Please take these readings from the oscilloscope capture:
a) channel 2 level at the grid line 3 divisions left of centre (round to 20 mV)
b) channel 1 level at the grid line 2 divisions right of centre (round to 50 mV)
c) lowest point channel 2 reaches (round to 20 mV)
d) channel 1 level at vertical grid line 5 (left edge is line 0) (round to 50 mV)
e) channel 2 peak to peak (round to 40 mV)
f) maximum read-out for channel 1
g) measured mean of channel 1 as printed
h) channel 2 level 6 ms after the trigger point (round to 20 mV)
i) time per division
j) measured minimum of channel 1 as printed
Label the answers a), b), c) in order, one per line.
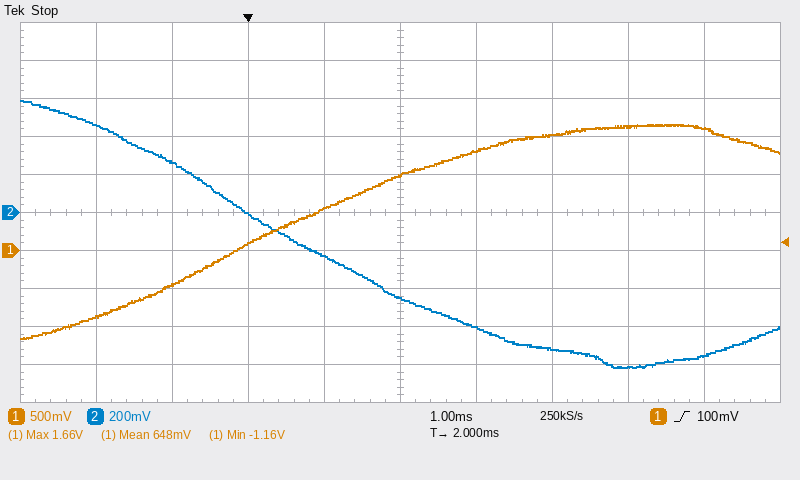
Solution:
a) 260 mV
b) 1.50 V
c) -820 mV
d) 1.00 V
e) 1.40 V
f) 1.66 V
g) 648 mV
h) -760 mV
i) 1 ms
j) -1.16 V
